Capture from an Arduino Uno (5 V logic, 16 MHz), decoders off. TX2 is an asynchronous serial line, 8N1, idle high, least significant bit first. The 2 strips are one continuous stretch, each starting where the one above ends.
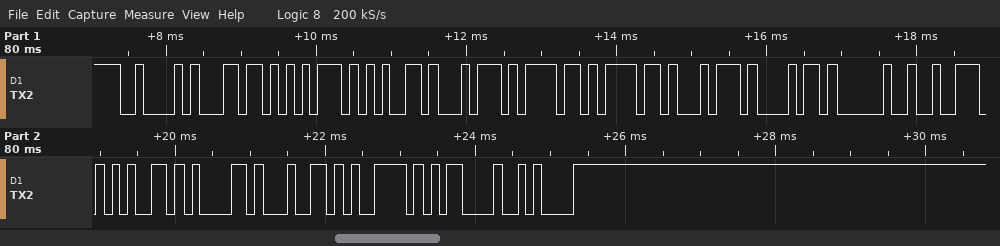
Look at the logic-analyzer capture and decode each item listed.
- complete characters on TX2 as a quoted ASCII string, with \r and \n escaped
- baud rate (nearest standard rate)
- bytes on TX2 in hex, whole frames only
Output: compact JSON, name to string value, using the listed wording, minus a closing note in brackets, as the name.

{"complete characters on TX2 as a quoted ASCII string, with \\r and \\n escaped": "\"Bluetooth ready\\r\\n\"", "baud rate": "9600 baud", "bytes on TX2 in hex, whole frames only": "42 6C 75 65 74 6F 6F 74 68 20 72 65 61 64 79 0D 0A"}
